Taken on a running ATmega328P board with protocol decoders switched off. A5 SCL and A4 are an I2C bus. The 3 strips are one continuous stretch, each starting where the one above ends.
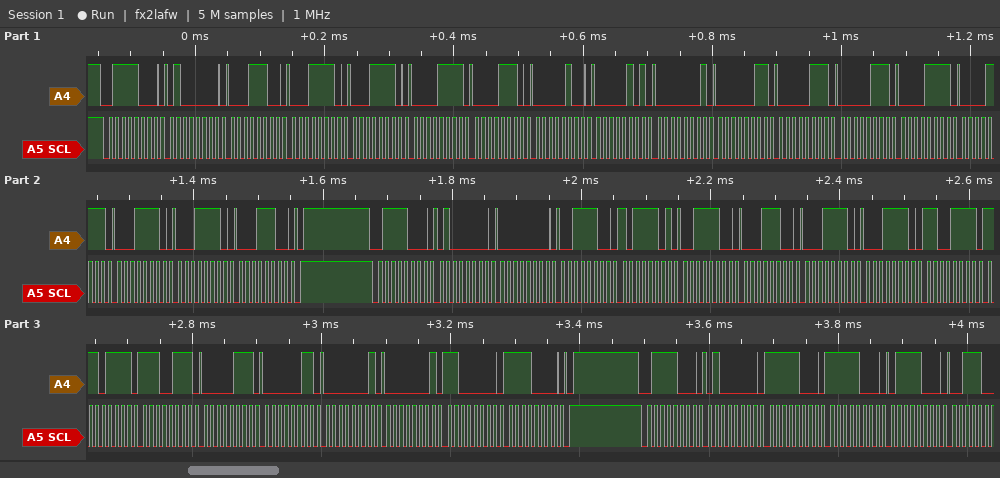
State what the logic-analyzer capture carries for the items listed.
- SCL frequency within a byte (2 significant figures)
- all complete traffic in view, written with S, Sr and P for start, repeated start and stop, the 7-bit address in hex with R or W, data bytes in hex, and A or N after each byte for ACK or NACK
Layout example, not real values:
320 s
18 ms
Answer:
100 kHz
S 3CW A 40 A 1C A 1E A 1E A 0F A 0E A 04 A 05 A 01 A 03 A 07 A 07 A 0F A 0F A 1E A 1E A 1C A P S 3CW A 40 A 00 A 3C A BD A 3C A 1C A 1E A 1E A CF A EF A E7 A 07 A 03 A 01 A 01 A C0 A F0 A P S 3CW A 40 A F8 A F8 A 78 A
